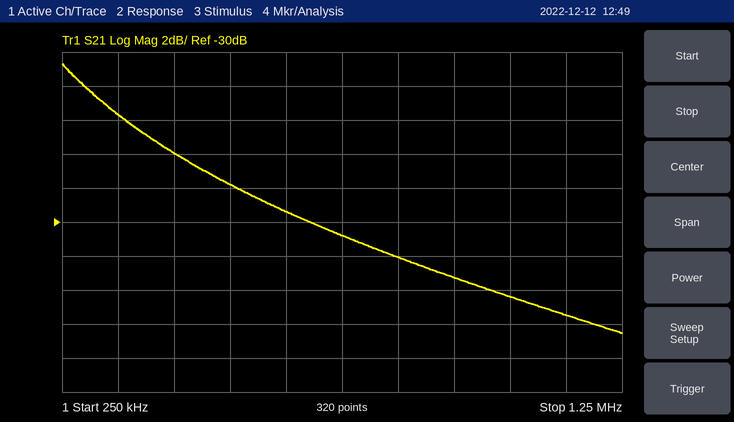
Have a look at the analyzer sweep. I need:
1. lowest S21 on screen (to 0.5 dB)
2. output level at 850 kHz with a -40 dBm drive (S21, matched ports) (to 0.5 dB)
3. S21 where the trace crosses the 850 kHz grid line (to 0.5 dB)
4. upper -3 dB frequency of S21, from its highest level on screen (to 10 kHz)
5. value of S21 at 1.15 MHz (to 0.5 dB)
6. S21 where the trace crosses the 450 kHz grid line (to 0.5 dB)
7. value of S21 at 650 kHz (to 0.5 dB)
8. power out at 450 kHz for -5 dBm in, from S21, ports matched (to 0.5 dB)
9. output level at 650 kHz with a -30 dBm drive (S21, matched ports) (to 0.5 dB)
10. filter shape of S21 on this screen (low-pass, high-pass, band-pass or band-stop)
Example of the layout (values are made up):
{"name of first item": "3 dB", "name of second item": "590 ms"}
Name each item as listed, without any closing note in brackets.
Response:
{"lowest S21 on screen": "-36.5 dB", "output level at 850 kHz with a -40 dBm drive (S21, matched ports)": "-72.0 dBm", "S21 where the trace crosses the 850 kHz grid line": "-32.0 dB", "upper -3 dB frequency of S21, from its highest level on screen": "350 kHz", "value of S21 at 1.15 MHz": "-35.5 dB", "S21 where the trace crosses the 450 kHz grid line": "-26.0 dB", "value of S21 at 650 kHz": "-29.5 dB", "power out at 450 kHz for -5 dBm in, from S21, ports matched": "-31.0 dBm", "output level at 650 kHz with a -30 dBm drive (S21, matched ports)": "-59.5 dBm", "filter shape of S21 on this screen": "low-pass"}
